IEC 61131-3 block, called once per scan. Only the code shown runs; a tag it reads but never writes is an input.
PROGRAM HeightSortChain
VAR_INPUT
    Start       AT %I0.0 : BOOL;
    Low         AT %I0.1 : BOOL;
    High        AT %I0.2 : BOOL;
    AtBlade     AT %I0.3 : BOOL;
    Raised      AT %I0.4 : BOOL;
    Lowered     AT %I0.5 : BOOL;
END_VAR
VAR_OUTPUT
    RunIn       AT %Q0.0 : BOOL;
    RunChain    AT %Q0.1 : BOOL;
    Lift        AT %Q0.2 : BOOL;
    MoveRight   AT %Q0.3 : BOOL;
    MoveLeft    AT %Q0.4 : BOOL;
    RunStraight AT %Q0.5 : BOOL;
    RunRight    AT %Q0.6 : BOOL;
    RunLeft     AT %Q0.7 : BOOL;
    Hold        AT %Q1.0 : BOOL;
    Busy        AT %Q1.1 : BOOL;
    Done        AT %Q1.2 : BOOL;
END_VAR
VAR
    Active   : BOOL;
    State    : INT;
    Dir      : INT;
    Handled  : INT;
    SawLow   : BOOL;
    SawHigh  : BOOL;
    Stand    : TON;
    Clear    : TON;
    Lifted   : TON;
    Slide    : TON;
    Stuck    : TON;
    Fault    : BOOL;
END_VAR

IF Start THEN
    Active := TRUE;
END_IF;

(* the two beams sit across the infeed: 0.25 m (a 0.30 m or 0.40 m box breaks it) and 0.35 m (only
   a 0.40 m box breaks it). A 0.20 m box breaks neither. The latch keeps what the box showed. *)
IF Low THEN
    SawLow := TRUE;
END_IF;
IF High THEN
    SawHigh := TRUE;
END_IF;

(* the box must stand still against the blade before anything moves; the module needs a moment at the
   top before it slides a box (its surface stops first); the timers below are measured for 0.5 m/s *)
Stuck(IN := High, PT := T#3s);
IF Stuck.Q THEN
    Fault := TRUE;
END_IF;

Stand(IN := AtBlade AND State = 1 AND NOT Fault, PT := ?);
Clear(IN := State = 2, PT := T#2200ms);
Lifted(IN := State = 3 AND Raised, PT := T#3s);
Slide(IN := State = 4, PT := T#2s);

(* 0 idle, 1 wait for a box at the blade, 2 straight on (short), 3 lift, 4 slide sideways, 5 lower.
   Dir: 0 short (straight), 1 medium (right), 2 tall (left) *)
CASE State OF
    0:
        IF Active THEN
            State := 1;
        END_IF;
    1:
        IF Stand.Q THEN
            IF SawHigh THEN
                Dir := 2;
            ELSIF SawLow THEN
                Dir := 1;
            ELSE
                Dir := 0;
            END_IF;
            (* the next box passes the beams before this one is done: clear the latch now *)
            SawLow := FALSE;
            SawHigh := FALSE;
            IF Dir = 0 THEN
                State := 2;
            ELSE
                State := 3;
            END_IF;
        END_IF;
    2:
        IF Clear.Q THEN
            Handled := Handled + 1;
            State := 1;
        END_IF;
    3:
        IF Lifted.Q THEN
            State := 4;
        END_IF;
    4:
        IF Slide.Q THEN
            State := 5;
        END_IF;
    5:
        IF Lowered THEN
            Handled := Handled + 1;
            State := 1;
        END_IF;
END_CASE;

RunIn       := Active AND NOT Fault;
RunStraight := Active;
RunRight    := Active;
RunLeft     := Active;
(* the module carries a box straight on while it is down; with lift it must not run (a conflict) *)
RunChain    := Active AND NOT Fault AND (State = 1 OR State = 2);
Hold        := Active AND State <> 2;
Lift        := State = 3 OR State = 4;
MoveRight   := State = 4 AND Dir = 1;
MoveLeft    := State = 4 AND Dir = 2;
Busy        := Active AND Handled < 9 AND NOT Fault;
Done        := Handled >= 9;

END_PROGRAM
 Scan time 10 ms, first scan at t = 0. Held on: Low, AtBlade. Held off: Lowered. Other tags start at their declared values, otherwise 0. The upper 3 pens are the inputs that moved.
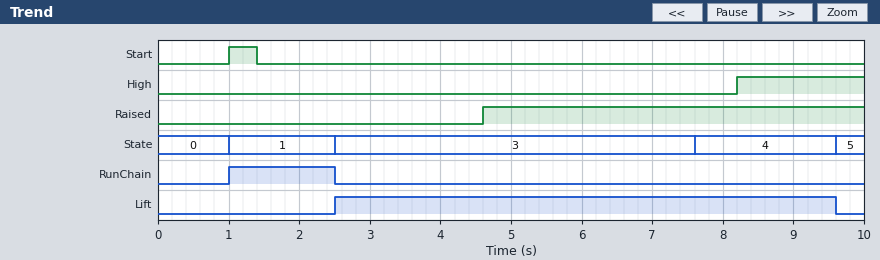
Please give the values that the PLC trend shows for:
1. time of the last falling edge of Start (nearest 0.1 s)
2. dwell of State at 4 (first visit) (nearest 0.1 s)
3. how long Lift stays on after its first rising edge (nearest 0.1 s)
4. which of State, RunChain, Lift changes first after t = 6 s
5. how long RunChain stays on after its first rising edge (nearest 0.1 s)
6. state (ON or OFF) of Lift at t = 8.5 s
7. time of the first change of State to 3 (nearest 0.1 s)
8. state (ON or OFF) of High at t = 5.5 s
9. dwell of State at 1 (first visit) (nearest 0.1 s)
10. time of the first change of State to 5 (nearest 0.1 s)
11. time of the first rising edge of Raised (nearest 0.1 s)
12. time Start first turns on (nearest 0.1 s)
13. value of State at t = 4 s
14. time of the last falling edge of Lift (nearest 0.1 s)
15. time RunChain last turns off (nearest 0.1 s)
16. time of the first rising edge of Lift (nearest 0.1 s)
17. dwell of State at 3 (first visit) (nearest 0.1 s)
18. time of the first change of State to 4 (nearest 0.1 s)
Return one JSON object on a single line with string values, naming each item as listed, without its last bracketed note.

{"time of the last falling edge of Start": "1.4 s", "dwell of State at 4 (first visit)": "2.0 s", "how long Lift stays on after its first rising edge": "7.1 s", "which of State, RunChain, Lift changes first after t = 6 s": "State", "how long RunChain stays on after its first rising edge": "1.5 s", "state (ON or OFF) of Lift at t = 8.5 s": "ON", "time of the first change of State to 3": "2.5 s", "state (ON or OFF) of High at t = 5.5 s": "OFF", "dwell of State at 1 (first visit)": "1.5 s", "time of the first change of State to 5": "9.6 s", "time of the first rising edge of Raised": "4.6 s", "time Start first turns on": "1.0 s", "value of State at t = 4 s": "3", "time of the last falling edge of Lift": "9.6 s", "time RunChain last turns off": "2.5 s", "time of the first rising edge of Lift": "2.5 s", "dwell of State at 3 (first visit)": "5.1 s", "time of the first change of State to 4": "7.6 s"}
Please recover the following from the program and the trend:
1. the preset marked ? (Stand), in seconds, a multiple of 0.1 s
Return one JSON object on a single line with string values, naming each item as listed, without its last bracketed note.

{"the preset marked ? (Stand), in seconds, a multiple of 0.1 s": "1.5 s"}
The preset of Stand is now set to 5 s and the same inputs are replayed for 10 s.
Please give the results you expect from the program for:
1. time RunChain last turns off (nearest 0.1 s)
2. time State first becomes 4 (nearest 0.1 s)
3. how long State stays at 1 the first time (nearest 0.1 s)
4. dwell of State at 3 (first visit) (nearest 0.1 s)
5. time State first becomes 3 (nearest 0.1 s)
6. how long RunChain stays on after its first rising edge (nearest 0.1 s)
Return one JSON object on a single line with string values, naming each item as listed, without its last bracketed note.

{"time RunChain last turns off": "6.0 s", "time State first becomes 4": "9.0 s", "how long State stays at 1 the first time": "5.0 s", "dwell of State at 3 (first visit)": "3.0 s", "time State first becomes 3": "6.0 s", "how long RunChain stays on after its first rising edge": "5.0 s"}
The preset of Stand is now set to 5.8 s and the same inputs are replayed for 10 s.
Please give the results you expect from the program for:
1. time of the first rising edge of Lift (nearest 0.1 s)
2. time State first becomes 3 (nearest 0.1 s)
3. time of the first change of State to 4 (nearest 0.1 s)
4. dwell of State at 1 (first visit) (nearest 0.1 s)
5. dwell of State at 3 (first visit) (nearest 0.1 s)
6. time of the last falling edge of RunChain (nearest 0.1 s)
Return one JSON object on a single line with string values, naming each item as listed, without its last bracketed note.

{"time of the first rising edge of Lift": "6.8 s", "time State first becomes 3": "6.8 s", "time of the first change of State to 4": "9.8 s", "dwell of State at 1 (first visit)": "5.8 s", "dwell of State at 3 (first visit)": "3.0 s", "time of the last falling edge of RunChain": "6.8 s"}
